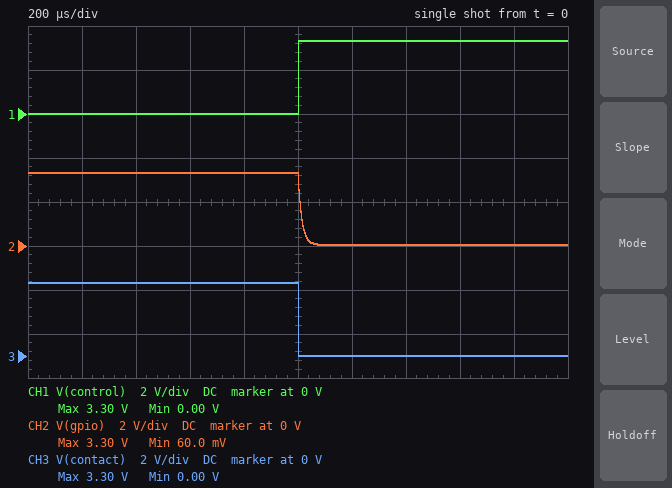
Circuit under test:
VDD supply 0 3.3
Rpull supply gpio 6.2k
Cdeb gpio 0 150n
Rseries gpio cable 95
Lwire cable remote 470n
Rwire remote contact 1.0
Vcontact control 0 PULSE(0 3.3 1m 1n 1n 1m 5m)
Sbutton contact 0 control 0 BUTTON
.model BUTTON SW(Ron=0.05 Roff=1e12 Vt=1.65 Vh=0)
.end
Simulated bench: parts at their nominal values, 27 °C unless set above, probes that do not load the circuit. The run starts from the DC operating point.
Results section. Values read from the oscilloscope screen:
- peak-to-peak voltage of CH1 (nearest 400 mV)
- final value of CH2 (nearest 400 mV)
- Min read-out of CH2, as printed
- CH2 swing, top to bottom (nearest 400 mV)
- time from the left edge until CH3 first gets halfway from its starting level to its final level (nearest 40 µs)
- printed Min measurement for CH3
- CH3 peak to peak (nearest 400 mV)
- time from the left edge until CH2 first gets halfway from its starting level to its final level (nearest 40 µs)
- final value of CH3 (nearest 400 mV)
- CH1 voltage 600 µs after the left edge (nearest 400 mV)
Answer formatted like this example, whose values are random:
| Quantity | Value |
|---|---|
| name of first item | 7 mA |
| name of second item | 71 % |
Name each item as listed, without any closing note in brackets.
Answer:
| Quantity | Value |
|---|---|
| peak-to-peak voltage of CH1 | 3.2 V |
| final value of CH2 | 0 V |
| Min read-out of CH2, as printed | 60.0 mV |
| CH2 swing, top to bottom | 3.2 V |
| time from the left edge until CH3 first gets halfway from its starting level to its final level | 1.00 ms |
| printed Min measurement for CH3 | 0.00 V |
| CH3 peak to peak | 3.2 V |
| time from the left edge until CH2 first gets halfway from its starting level to its final level | 1.00 ms |
| final value of CH3 | 0 V |
| CH1 voltage 600 µs after the left edge | 0 V |
